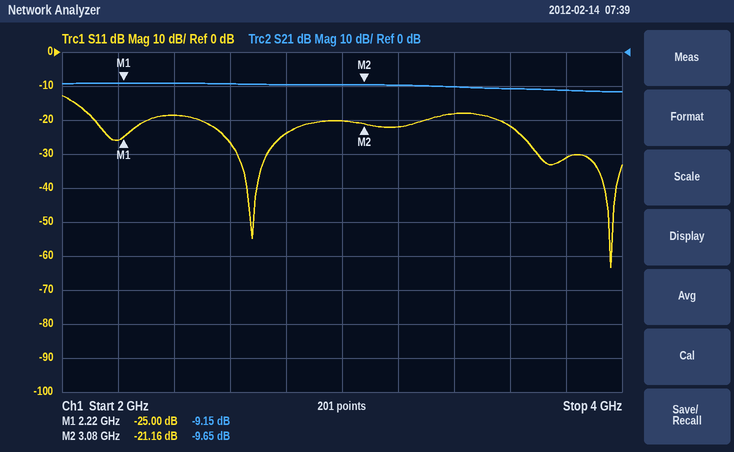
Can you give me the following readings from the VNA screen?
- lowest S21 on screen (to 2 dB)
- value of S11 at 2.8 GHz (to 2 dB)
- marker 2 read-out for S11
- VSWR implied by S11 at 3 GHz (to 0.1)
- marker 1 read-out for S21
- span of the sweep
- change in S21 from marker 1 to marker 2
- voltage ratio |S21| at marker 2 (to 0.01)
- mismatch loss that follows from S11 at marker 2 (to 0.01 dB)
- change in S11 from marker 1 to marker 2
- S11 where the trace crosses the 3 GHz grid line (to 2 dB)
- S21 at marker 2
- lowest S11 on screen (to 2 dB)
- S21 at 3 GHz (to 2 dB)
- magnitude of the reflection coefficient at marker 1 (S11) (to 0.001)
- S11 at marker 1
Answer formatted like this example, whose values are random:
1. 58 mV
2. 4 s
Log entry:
1. -12 dB
2. -24 dB
3. -21.16 dB
4. 1.2
5. -9.15 dB
6. 2 GHz
7. -0.50 dB
8. 0.33
9. 0.03 dB
10. 3.84 dB
11. -20 dB
12. -9.65 dB
13. -64 dB
14. -10 dB
15. 0.056
16. -25.00 dB
